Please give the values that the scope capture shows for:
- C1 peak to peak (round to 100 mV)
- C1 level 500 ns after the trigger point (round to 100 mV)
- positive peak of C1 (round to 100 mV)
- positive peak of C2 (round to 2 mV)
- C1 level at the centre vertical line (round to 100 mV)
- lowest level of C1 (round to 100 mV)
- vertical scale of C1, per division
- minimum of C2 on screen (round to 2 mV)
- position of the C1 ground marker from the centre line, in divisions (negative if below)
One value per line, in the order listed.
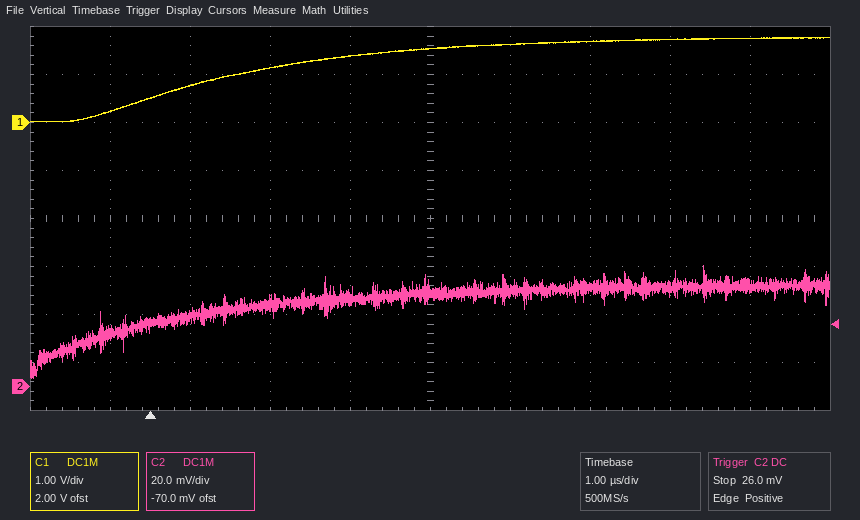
1.8 V
800 mV
1.8 V
50 mV
1.5 V
0.0 V
1 V
4 mV
+2.0 div
